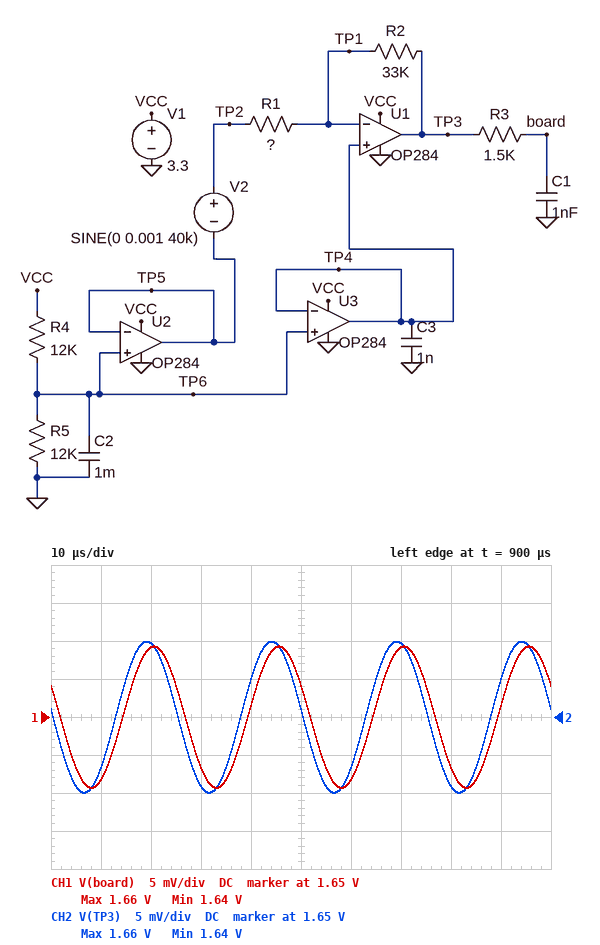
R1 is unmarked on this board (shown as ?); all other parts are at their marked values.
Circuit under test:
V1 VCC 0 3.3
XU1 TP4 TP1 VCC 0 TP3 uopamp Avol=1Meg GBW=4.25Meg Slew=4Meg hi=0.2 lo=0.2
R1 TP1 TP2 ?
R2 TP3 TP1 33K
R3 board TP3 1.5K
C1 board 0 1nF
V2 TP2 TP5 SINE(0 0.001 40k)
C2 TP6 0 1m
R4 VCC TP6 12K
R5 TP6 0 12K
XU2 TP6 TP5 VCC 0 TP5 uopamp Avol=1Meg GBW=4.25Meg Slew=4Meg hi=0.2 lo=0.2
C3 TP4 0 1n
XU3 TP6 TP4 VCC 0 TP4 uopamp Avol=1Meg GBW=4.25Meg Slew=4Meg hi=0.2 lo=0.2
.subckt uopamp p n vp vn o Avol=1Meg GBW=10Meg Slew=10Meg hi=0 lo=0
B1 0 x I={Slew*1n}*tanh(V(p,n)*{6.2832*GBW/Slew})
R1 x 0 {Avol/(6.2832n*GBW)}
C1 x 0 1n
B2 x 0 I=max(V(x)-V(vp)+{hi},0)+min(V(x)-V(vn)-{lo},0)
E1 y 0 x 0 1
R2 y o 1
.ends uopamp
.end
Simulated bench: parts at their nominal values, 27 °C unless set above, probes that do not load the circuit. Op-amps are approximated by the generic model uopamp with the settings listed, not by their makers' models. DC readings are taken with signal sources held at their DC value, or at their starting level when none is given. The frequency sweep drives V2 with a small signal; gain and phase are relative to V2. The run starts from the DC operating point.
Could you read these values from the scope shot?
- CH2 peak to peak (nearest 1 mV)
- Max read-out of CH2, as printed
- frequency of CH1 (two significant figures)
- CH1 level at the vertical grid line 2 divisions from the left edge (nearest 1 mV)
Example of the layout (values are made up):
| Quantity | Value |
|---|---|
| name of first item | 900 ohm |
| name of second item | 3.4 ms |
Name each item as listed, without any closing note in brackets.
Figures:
| Quantity | Value |
|---|---|
| CH2 peak to peak | 20 mV |
| Max read-out of CH2, as printed | 1.66 V |
| frequency of CH1 | 40 kHz |
| CH1 level at the vertical grid line 2 divisions from the left edge | 1.659 V |
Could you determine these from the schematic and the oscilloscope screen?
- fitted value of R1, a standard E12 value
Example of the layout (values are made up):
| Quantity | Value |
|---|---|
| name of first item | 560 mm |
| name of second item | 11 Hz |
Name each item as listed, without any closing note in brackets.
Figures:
| Quantity | Value |
|---|---|
| fitted value of R1, a standard E12 value | 3.3 kΩ |
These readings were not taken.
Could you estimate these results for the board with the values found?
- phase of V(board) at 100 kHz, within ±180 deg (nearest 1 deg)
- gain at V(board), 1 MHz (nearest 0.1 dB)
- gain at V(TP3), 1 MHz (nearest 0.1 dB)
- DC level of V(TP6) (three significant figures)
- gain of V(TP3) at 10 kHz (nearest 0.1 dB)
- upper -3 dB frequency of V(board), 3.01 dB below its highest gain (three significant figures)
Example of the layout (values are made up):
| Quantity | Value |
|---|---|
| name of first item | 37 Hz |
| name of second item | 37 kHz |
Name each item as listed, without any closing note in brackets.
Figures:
| Quantity | Value |
|---|---|
| phase of V(board) at 100 kHz, within ±180 deg | 122 deg |
| gain at V(board), 1 MHz | -8.4 dB |
| gain at V(TP3), 1 MHz | 11.1 dB |
| DC level of V(TP6) | 1.65 V |
| gain of V(TP3) at 10 kHz | 20.0 dB |
| upper -3 dB frequency of V(board), 3.01 dB below its highest gain | 99.3 kHz |
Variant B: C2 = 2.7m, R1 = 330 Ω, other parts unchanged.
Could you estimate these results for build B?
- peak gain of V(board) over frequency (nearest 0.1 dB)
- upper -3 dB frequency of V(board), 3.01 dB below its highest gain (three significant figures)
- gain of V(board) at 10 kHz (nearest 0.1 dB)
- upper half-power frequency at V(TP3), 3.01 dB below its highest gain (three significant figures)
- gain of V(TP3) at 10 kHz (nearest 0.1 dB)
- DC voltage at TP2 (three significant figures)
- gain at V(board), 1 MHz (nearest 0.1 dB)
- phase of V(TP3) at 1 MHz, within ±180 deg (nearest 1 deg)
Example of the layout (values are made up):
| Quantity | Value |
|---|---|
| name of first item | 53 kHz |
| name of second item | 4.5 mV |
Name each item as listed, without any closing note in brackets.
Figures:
| Quantity | Value |
|---|---|
| peak gain of V(board) over frequency | 40.0 dB |
| upper -3 dB frequency of V(board), 3.01 dB below its highest gain | 37.2 kHz |
| gain of V(board) at 10 kHz | 39.7 dB |
| upper half-power frequency at V(TP3), 3.01 dB below its highest gain | 42.1 kHz |
| gain of V(TP3) at 10 kHz | 39.8 dB |
| DC voltage at TP2 | 1.65 V |
| gain at V(board), 1 MHz | -7.1 dB |
| phase of V(TP3) at 1 MHz, within ±180 deg | 92 deg |
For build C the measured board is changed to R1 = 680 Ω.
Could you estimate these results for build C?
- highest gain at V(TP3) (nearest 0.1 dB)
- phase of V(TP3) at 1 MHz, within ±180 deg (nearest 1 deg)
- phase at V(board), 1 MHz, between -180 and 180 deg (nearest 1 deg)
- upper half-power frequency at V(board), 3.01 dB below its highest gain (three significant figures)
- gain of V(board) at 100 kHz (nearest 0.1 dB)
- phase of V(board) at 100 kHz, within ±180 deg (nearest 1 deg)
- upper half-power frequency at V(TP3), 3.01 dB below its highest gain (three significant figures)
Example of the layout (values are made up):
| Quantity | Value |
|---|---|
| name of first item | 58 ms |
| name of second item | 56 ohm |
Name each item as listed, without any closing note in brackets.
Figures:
| Quantity | Value |
|---|---|
| highest gain at V(TP3) | 33.7 dB |
| phase of V(TP3) at 1 MHz, within ±180 deg | 95 deg |
| phase at V(board), 1 MHz, between -180 and 180 deg | 11 deg |
| upper half-power frequency at V(board), 3.01 dB below its highest gain | 60.9 kHz |
| gain of V(board) at 100 kHz | 27.2 dB |
| phase of V(board) at 100 kHz, within ±180 deg | 87 deg |
| upper half-power frequency at V(TP3), 3.01 dB below its highest gain | 85.8 kHz |
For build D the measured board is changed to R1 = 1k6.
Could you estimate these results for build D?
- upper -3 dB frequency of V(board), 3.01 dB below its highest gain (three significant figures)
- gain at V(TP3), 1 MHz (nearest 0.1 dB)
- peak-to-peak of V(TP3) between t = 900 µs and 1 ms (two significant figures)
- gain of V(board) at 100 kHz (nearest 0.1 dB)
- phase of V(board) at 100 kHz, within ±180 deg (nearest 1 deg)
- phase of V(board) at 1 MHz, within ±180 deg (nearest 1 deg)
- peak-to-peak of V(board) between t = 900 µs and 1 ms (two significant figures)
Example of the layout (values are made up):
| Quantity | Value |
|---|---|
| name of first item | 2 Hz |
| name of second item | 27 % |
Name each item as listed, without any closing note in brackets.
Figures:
| Quantity | Value |
|---|---|
| upper -3 dB frequency of V(board), 3.01 dB below its highest gain | 87.0 kHz |
| gain at V(TP3), 1 MHz | 12.0 dB |
| peak-to-peak of V(TP3) between t = 900 µs and 1 ms | 40 mV |
| gain of V(board) at 100 kHz | 22.5 dB |
| phase of V(board) at 100 kHz, within ±180 deg | 110 deg |
| phase of V(board) at 1 MHz, within ±180 deg | 17 deg |
| peak-to-peak of V(board) between t = 900 µs and 1 ms | 38 mV |
